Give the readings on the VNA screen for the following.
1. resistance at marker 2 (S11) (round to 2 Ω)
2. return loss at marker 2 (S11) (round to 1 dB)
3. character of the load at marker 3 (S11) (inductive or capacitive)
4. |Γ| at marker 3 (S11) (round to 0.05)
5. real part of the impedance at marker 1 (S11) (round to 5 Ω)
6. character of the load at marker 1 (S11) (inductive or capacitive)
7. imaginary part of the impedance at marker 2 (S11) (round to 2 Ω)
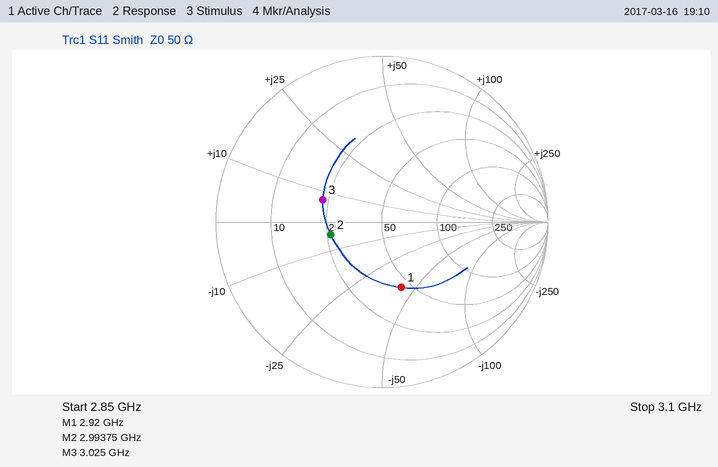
26 Ω
10 dB
inductive
0.40
45 Ω
capacitive
-4 Ω
